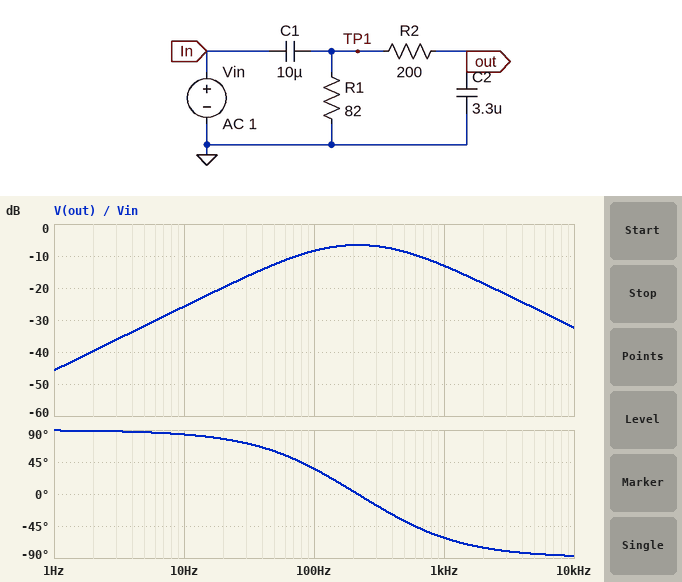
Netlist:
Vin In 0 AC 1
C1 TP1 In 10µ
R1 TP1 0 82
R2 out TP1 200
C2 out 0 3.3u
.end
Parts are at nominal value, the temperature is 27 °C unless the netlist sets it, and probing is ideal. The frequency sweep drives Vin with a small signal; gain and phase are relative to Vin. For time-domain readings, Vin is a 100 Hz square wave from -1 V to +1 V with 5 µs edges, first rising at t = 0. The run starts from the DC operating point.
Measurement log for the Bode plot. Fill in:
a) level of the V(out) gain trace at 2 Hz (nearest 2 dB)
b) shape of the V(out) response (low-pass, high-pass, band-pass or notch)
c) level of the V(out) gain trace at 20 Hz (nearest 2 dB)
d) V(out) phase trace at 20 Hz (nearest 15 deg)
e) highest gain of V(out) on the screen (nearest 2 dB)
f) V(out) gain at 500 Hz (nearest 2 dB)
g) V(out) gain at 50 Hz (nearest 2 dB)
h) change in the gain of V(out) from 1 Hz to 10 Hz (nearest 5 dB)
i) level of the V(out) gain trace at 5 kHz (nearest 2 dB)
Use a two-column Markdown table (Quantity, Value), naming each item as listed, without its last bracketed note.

| Quantity | Value |
|---|---|
| level of the V(out) gain trace at 2 Hz | -40 dB |
| shape of the V(out) response | band-pass |
| level of the V(out) gain trace at 20 Hz | -20 dB |
| V(out) phase trace at 20 Hz | 75 deg |
| highest gain of V(out) on the screen | -6 dB |
| V(out) gain at 500 Hz | -8 dB |
| V(out) gain at 50 Hz | -12 dB |
| change in the gain of V(out) from 1 Hz to 10 Hz | 20 dB |
| level of the V(out) gain trace at 5 kHz | -26 dB |
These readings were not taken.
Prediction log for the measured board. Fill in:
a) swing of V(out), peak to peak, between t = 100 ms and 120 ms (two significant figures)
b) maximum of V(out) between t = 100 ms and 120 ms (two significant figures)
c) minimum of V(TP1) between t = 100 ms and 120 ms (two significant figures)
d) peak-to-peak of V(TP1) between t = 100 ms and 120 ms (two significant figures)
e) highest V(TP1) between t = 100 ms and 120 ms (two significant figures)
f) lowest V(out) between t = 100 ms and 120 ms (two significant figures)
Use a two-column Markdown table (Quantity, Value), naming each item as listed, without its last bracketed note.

| Quantity | Value |
|---|---|
| swing of V(out), peak to peak, between t = 100 ms and 120 ms | 1.4 V |
| maximum of V(out) between t = 100 ms and 120 ms | 700 mV |
| minimum of V(TP1) between t = 100 ms and 120 ms | -2.0 V |
| peak-to-peak of V(TP1) between t = 100 ms and 120 ms | 3.9 V |
| highest V(TP1) between t = 100 ms and 120 ms | 2.0 V |
| lowest V(out) between t = 100 ms and 120 ms | -700 mV |
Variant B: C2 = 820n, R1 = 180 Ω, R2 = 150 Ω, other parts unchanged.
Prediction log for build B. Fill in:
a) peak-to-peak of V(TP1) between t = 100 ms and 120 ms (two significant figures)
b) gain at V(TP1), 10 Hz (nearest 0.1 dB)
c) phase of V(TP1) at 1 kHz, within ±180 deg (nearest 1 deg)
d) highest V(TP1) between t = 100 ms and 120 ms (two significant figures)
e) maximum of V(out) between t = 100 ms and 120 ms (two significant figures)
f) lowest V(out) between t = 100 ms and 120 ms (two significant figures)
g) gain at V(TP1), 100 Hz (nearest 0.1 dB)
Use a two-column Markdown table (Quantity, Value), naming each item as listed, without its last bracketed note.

| Quantity | Value |
|---|---|
| peak-to-peak of V(TP1) between t = 100 ms and 120 ms | 3.7 V |
| gain at V(TP1), 10 Hz | -19.0 dB |
| phase of V(TP1) at 1 kHz, within ±180 deg | 7 deg |
| highest V(TP1) between t = 100 ms and 120 ms | 1.9 V |
| maximum of V(out) between t = 100 ms and 120 ms | 1.4 V |
| lowest V(out) between t = 100 ms and 120 ms | -1.4 V |
| gain at V(TP1), 100 Hz | -2.9 dB |
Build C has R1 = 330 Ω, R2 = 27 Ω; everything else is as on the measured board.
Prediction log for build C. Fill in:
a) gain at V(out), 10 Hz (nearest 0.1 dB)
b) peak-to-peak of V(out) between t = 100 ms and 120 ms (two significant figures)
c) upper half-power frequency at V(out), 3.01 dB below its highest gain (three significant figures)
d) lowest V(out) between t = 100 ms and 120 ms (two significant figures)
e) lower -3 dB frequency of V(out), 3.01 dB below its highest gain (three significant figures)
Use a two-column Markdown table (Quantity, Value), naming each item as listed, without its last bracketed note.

| Quantity | Value |
|---|---|
| gain at V(out), 10 Hz | -14.0 dB |
| peak-to-peak of V(out) between t = 100 ms and 120 ms | 2.1 V |
| upper half-power frequency at V(out), 3.01 dB below its highest gain | 2.46 kHz |
| lowest V(out) between t = 100 ms and 120 ms | -1.1 V |
| lower -3 dB frequency of V(out), 3.01 dB below its highest gain | 35.0 Hz |
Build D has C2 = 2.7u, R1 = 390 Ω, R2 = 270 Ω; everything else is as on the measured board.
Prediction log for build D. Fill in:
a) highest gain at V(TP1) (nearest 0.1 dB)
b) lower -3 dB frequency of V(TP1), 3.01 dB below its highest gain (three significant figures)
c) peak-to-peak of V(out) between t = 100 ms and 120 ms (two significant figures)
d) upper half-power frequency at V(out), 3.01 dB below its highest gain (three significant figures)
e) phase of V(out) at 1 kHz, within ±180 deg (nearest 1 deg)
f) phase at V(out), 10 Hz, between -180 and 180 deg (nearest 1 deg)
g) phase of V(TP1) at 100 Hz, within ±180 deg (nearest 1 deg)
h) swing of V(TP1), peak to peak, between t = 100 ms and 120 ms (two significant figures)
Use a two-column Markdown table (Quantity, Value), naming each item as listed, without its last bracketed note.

| Quantity | Value |
|---|---|
| highest gain at V(TP1) | 0 dB |
| lower -3 dB frequency of V(TP1), 3.01 dB below its highest gain | 68.9 Hz |
| peak-to-peak of V(out) between t = 100 ms and 120 ms | 1.6 V |
| upper half-power frequency at V(out), 3.01 dB below its highest gain | 344 Hz |
| phase of V(out) at 1 kHz, within ±180 deg | -72 deg |
| phase at V(out), 10 Hz, between -180 and 180 deg | 70 deg |
| phase of V(TP1) at 100 Hz, within ±180 deg | 23 deg |
| swing of V(TP1), peak to peak, between t = 100 ms and 120 ms | 3.2 V |
